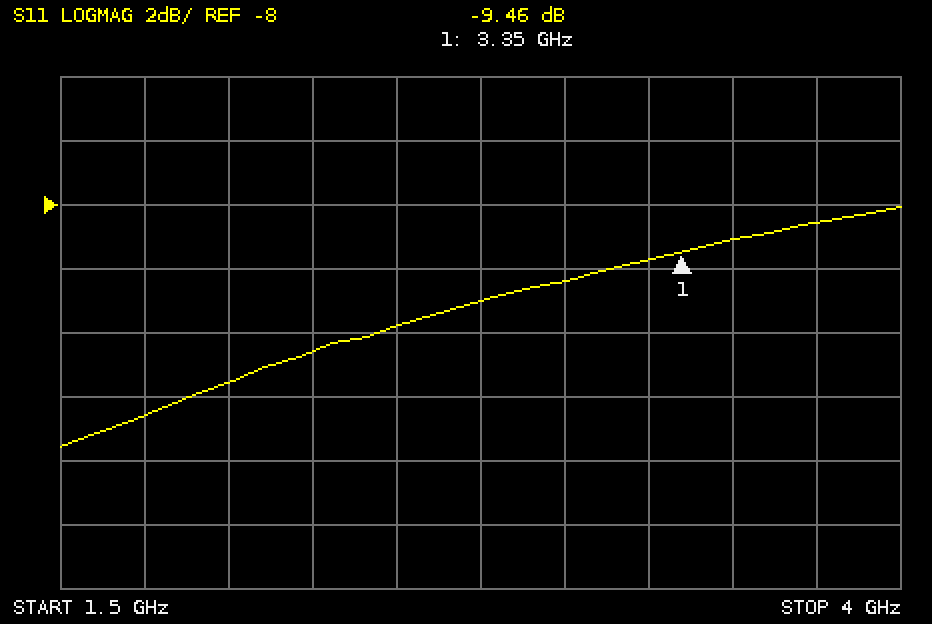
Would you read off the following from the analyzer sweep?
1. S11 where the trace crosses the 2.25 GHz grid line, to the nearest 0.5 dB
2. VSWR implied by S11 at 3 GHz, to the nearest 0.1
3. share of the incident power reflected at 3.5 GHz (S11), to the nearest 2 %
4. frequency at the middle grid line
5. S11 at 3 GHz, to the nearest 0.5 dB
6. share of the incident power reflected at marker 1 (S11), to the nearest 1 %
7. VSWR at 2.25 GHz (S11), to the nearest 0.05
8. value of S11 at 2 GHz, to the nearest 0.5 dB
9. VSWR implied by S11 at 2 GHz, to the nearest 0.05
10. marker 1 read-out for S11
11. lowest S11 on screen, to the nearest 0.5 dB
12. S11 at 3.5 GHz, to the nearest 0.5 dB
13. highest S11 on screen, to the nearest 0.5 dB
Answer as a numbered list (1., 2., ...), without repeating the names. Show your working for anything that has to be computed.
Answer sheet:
1. -12.5 dB
2. |Γ| = 10^(-10.5/20) = 0.2985; VSWR = (1 + 0.2985)/(1 − 0.2985) ≈ 1.9
3. 10^(-9/10) ≈ 12.6 %, so 12 % to the nearest 2 %
4. 2.75 GHz
5. -10.5 dB
6. 10^(-9.46/10) ≈ 11 %
7. |Γ| = 10^(-12.5/20) = 0.2371; VSWR = (1 + 0.2371)/(1 − 0.2371) ≈ 1.62, so 1.60 to the nearest 0.05
8. -13.5 dB
9. |Γ| = 10^(-13.5/20) = 0.2113; VSWR = (1 + 0.2113)/(1 − 0.2113) ≈ 1.54, so 1.55 to the nearest 0.05
10. -9.46 dB
11. -15.5 dB
12. -9.0 dB
13. -8.0 dB
